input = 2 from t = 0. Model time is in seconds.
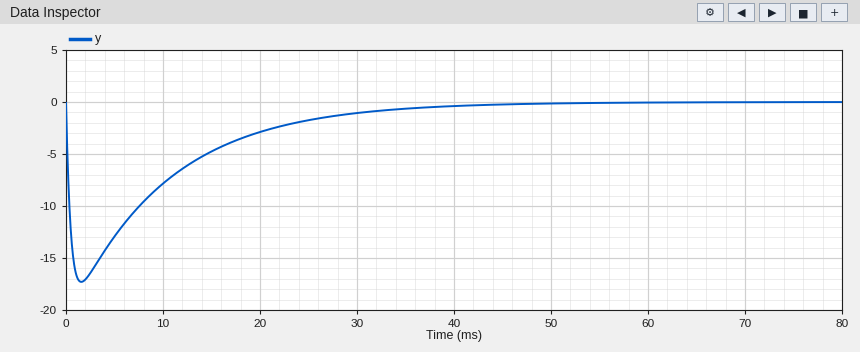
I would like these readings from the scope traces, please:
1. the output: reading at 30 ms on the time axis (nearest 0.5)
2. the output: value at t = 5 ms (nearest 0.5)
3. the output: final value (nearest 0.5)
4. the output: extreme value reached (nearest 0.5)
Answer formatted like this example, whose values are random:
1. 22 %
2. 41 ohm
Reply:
1. -1.0
2. -13.0
3. 0.0
4. -17.5
